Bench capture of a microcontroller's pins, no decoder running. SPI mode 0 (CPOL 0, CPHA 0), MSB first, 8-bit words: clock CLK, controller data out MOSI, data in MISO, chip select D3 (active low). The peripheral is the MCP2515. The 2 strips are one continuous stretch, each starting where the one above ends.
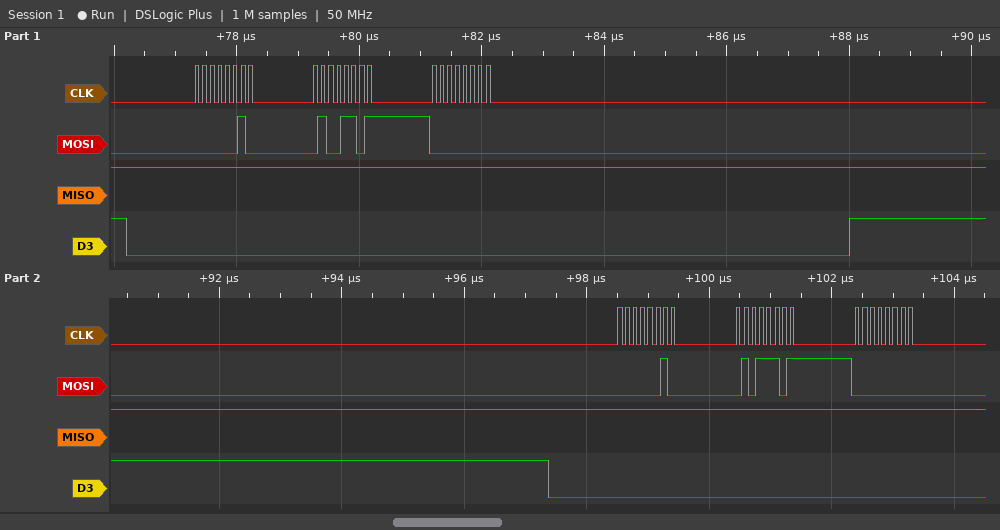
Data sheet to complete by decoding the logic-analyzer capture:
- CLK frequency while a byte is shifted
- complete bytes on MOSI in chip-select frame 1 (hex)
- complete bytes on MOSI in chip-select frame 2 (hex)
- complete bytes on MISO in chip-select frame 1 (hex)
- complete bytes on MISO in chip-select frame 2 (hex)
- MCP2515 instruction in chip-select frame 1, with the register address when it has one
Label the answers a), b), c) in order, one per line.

a) 8 MHz
b) 02 4D 00
c) 02 5D 00
d) FF FF FF
e) FF FF FF
f) WRITE 0x4D
